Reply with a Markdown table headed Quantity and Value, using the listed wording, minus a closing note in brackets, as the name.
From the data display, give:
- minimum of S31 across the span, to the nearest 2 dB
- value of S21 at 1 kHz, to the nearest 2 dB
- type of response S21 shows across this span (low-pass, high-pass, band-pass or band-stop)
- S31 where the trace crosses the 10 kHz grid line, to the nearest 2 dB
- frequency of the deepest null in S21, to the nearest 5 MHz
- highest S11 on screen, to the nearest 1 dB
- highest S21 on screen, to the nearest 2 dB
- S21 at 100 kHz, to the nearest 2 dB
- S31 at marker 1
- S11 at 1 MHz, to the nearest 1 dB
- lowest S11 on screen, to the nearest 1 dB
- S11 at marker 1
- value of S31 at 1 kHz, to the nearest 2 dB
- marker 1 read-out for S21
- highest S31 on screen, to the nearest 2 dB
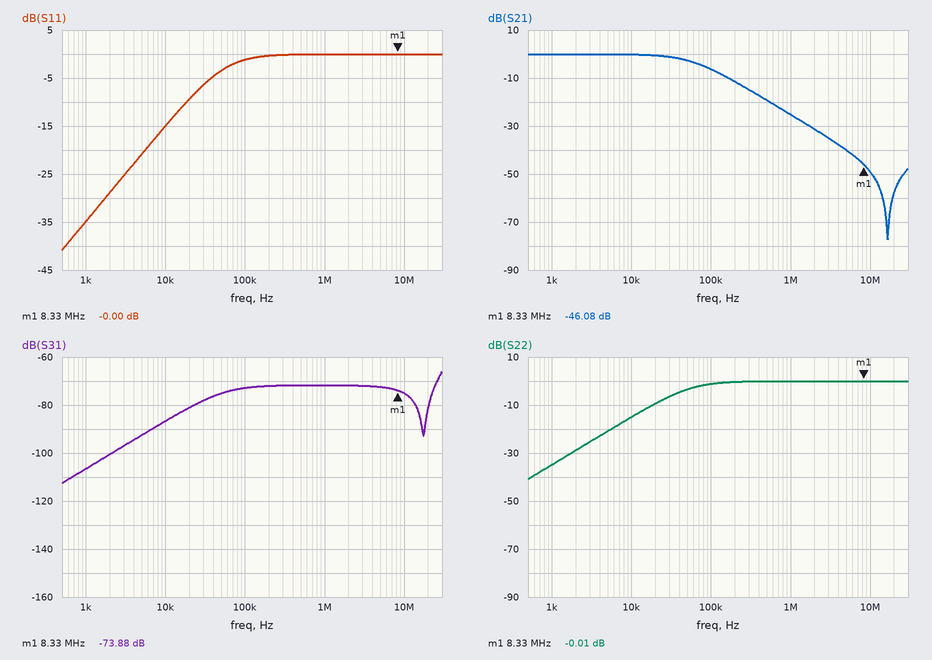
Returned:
| Quantity | Value |
|---|---|
| minimum of S31 across the span, to the nearest 2 dB | -112 dB |
| value of S21 at 1 kHz, to the nearest 2 dB | 0 dB |
| type of response S21 shows across this span | low-pass |
| S31 where the trace crosses the 10 kHz grid line, to the nearest 2 dB | -86 dB |
| frequency of the deepest null in S21, to the nearest 5 MHz | 15 MHz |
| highest S11 on screen, to the nearest 1 dB | 0 dB |
| highest S21 on screen, to the nearest 2 dB | 0 dB |
| S21 at 100 kHz, to the nearest 2 dB | -6 dB |
| S31 at marker 1 | -73.88 dB |
| S11 at 1 MHz, to the nearest 1 dB | 0 dB |
| lowest S11 on screen, to the nearest 1 dB | -41 dB |
| S11 at marker 1 | -0.00 dB |
| value of S31 at 1 kHz, to the nearest 2 dB | -106 dB |
| marker 1 read-out for S21 | -46.08 dB |
| highest S31 on screen, to the nearest 2 dB | -66 dB |
